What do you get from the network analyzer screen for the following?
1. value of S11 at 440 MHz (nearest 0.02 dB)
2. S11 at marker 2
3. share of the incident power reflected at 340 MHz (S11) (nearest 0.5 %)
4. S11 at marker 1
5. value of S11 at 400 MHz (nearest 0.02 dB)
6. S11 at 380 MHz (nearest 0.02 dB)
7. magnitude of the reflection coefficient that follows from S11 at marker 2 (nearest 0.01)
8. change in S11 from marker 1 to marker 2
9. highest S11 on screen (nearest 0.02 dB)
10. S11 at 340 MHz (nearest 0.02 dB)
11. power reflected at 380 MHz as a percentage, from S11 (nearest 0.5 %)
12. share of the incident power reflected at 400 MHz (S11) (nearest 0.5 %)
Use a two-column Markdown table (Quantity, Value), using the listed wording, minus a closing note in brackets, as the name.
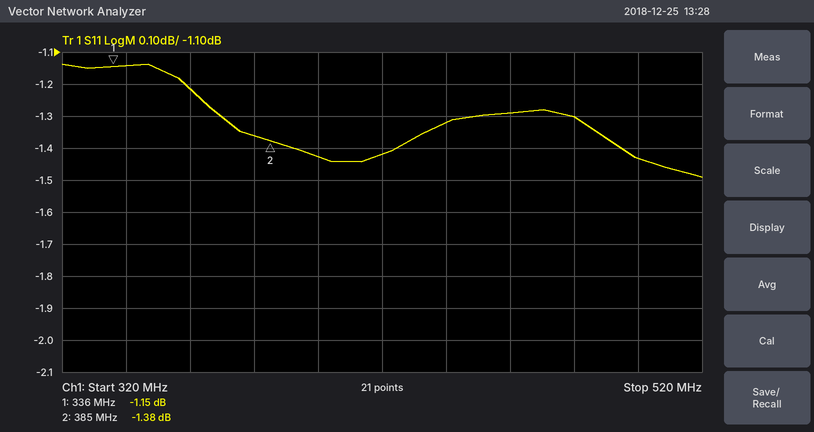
| Quantity | Value |
|---|---|
| value of S11 at 440 MHz | -1.32 dB |
| S11 at marker 2 | -1.38 dB |
| share of the incident power reflected at 340 MHz (S11) | 77.0 % |
| S11 at marker 1 | -1.15 dB |
| value of S11 at 400 MHz | -1.42 dB |
| S11 at 380 MHz | -1.36 dB |
| magnitude of the reflection coefficient that follows from S11 at marker 2 | 0.85 |
| change in S11 from marker 1 to marker 2 | -0.23 dB |
| highest S11 on screen | -1.14 dB |
| S11 at 340 MHz | -1.14 dB |
| power reflected at 380 MHz as a percentage, from S11 | 73.0 % |
| share of the incident power reflected at 400 MHz (S11) | 72.0 % |
